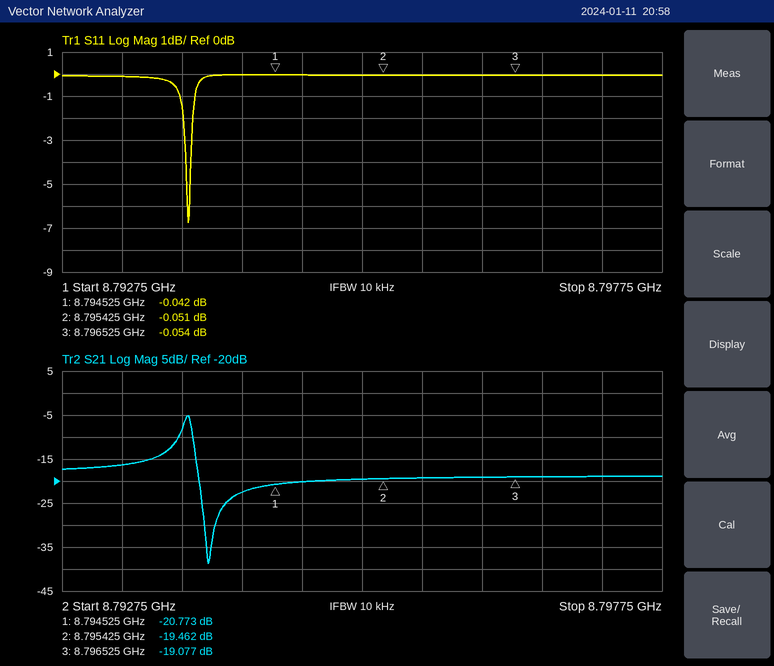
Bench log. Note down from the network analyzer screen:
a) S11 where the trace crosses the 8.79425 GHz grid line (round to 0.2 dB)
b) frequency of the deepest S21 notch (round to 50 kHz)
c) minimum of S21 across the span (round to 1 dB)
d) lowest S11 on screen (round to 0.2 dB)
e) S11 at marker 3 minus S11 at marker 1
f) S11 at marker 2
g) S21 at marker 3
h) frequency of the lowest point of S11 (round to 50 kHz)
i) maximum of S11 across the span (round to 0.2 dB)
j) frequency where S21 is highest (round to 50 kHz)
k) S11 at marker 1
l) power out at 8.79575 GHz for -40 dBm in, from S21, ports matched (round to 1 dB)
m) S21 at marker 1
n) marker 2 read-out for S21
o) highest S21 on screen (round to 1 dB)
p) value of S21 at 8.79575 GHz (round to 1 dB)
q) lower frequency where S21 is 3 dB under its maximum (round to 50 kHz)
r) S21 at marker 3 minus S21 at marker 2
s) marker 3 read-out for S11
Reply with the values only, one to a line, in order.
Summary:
0.0 dB
8.79395 GHz
-39 dB
-6.8 dB
-0.012 dB
-0.051 dB
-19.077 dB
8.79380 GHz
0.0 dB
8.79380 GHz
-0.042 dB
-59 dBm
-20.773 dB
-19.462 dB
-5 dB
-19 dB
8.79375 GHz
0.385 dB
-0.054 dB
